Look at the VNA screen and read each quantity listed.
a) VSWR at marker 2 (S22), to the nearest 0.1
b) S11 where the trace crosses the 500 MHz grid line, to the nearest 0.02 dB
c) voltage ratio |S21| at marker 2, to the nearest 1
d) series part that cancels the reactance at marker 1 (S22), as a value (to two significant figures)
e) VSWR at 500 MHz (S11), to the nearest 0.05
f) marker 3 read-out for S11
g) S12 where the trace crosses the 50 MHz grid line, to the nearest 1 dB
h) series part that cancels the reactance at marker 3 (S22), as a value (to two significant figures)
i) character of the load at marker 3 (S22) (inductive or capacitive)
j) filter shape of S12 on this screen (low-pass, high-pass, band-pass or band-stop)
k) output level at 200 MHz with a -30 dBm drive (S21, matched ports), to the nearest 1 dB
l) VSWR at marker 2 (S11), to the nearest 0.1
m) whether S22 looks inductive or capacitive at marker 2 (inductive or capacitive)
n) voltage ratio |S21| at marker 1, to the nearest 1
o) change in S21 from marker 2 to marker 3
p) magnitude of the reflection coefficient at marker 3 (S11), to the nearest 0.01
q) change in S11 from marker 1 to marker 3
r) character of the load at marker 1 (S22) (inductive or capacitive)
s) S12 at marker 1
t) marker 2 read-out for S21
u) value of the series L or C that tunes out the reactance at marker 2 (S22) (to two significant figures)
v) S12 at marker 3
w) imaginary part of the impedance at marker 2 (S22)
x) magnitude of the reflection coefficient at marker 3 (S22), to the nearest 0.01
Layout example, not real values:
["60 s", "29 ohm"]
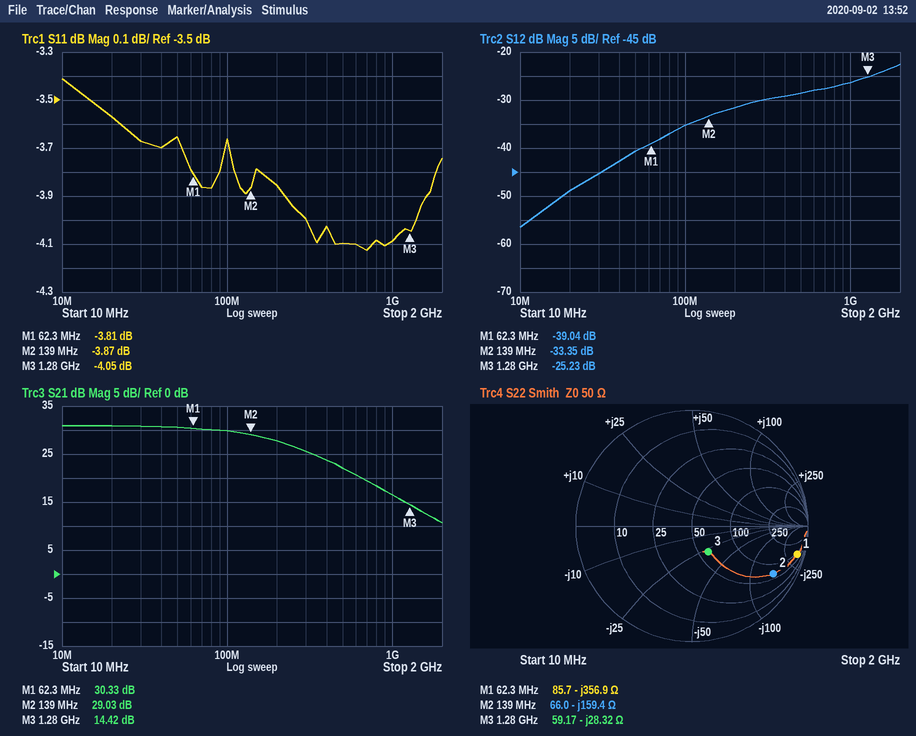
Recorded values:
["9.7", "-4.10 dB", "28", "910 nH", "4.30", "-4.05 dB", "-41 dB", "3.5 nH", "capacitive", "high-pass", "-2 dBm", "4.6", "capacitive", "33", "-14.61 dB", "0.63", "-0.24 dB", "capacitive", "-39.04 dB", "29.03 dB", "180 nH", "-25.23 dB", "-159.4 Ω", "0.26"]
